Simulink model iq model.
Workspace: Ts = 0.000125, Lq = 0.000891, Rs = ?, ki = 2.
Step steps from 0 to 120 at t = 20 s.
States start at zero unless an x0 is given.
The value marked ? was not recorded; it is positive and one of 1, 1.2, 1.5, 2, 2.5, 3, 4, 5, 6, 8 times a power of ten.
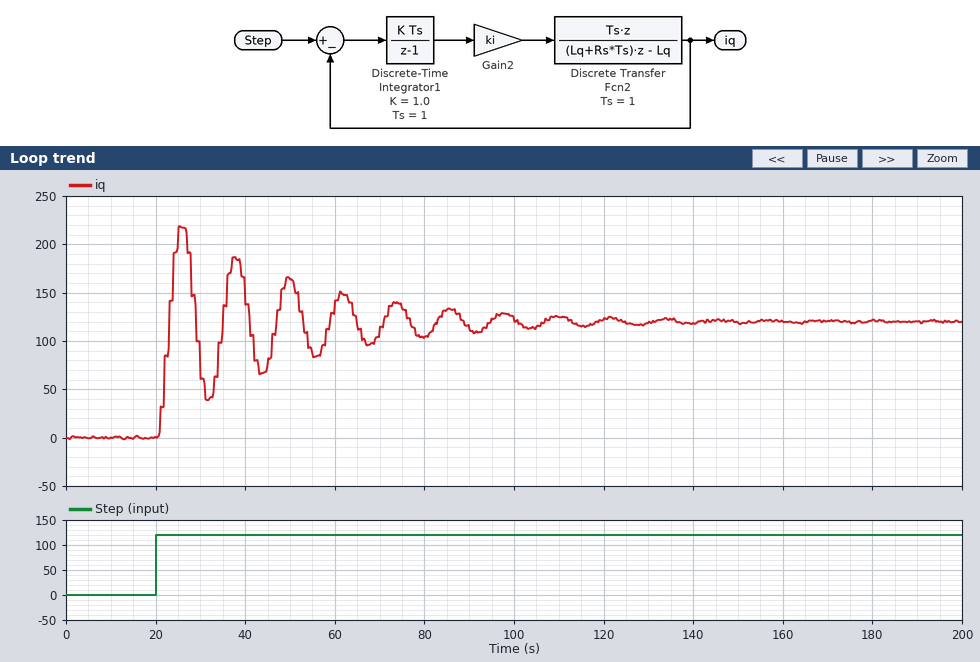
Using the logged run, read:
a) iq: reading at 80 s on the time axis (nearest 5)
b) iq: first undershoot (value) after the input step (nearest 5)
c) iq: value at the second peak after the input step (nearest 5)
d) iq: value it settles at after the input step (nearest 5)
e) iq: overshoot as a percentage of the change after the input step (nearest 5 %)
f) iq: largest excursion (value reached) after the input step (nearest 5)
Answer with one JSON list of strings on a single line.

["105", "40", "185", "120", "80 %", "220"]
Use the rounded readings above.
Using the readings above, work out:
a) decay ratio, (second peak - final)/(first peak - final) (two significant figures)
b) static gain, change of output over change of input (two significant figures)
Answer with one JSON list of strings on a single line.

["0.65", "1.0"]
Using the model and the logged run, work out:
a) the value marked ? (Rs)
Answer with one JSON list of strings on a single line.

["0.5"]
